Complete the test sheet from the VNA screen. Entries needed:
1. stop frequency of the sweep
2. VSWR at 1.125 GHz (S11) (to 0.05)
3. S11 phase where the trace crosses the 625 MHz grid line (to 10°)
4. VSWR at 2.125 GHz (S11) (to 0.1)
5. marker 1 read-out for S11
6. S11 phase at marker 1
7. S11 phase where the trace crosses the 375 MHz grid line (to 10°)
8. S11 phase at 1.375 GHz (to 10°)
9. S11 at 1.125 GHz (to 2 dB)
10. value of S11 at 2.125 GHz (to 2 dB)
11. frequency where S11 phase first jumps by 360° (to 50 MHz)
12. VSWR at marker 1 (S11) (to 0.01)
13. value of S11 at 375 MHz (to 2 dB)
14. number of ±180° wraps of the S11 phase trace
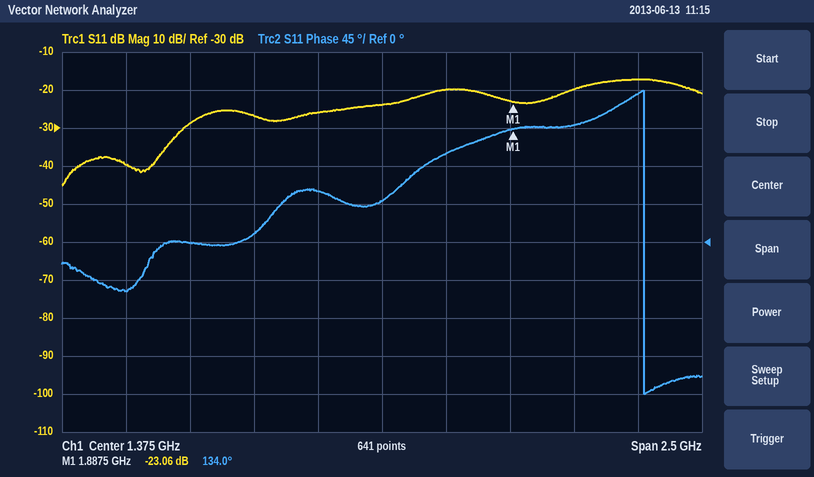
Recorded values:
2.625 GHz
1.10
0°
1.2
-23.06 dB
134.0°
-60°
50°
-26 dB
-20 dB
2.40 GHz
1.15
-40 dB
1
